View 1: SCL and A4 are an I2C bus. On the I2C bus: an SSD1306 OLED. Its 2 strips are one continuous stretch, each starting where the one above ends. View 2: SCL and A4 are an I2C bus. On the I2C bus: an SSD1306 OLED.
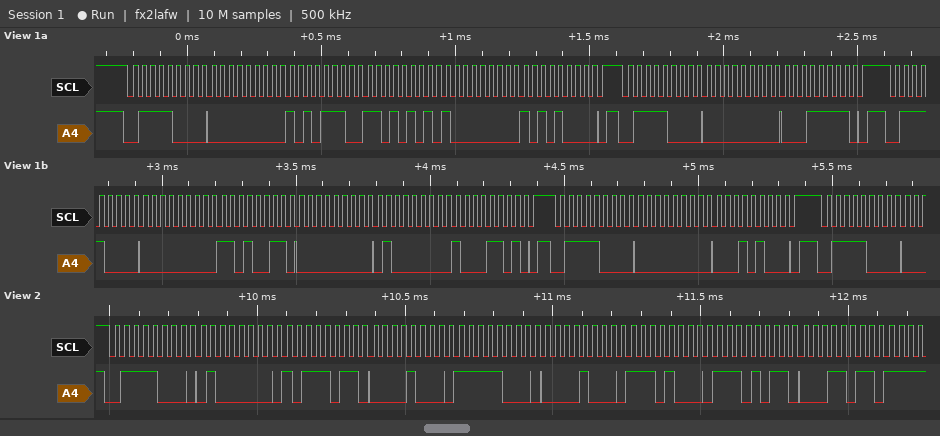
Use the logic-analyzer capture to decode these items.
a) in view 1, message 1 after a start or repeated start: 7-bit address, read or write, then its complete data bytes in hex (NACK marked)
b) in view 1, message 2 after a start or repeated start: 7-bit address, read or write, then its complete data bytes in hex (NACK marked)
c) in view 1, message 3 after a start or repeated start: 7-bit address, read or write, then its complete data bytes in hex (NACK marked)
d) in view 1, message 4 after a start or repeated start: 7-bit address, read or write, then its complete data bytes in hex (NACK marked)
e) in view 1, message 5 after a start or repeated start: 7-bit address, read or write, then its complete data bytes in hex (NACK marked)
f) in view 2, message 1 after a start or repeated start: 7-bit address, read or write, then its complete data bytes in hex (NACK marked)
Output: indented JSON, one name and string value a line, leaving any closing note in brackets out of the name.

{
  "in view 1, message 1 after a start or repeated start: 7-bit address, read or write, then its complete data bytes in hex": "0x3C write: 00 AE D5 80 A8",
  "in view 1, message 2 after a start or repeated start: 7-bit address, read or write, then its complete data bytes in hex": "0x3C write: 00 1F",
  "in view 1, message 3 after a start or repeated start: 7-bit address, read or write, then its complete data bytes in hex": "0x3C write: 00 D3 00 40 8D",
  "in view 1, message 4 after a start or repeated start: 7-bit address, read or write, then its complete data bytes in hex": "0x3C write: 00 14",
  "in view 1, message 5 after a start or repeated start: 7-bit address, read or write, then its complete data bytes in hex": "0x3C write",
  "in view 2, message 1 after a start or repeated start: 7-bit address, read or write, then its complete data bytes in hex": "0x3C write: 40 BB 08 F8 08 E8 EB 1B"
}
